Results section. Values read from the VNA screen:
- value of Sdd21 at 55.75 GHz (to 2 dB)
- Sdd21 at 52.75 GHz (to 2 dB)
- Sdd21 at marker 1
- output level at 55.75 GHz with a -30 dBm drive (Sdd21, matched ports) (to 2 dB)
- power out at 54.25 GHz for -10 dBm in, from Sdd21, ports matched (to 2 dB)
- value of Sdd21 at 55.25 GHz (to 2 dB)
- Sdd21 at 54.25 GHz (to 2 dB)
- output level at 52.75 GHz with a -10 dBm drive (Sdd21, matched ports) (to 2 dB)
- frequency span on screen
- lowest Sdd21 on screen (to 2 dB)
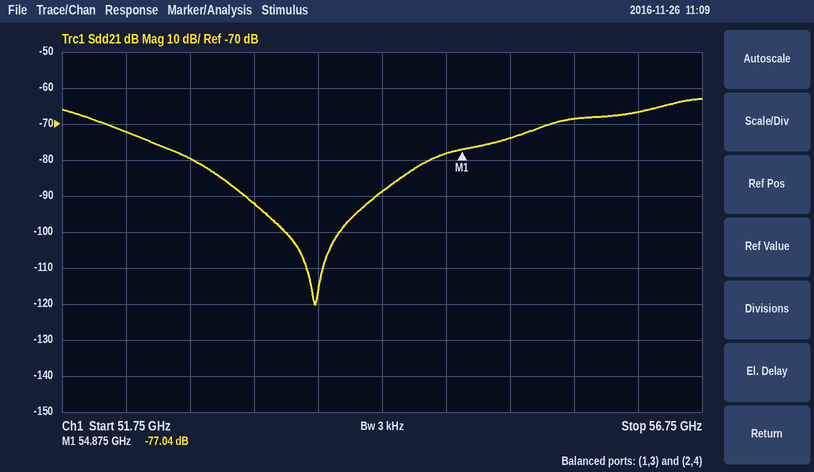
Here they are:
-68 dB
-80 dB
-77.04 dB
-98 dBm
-98 dBm
-74 dB
-88 dB
-90 dBm
5 GHz
-120 dB
